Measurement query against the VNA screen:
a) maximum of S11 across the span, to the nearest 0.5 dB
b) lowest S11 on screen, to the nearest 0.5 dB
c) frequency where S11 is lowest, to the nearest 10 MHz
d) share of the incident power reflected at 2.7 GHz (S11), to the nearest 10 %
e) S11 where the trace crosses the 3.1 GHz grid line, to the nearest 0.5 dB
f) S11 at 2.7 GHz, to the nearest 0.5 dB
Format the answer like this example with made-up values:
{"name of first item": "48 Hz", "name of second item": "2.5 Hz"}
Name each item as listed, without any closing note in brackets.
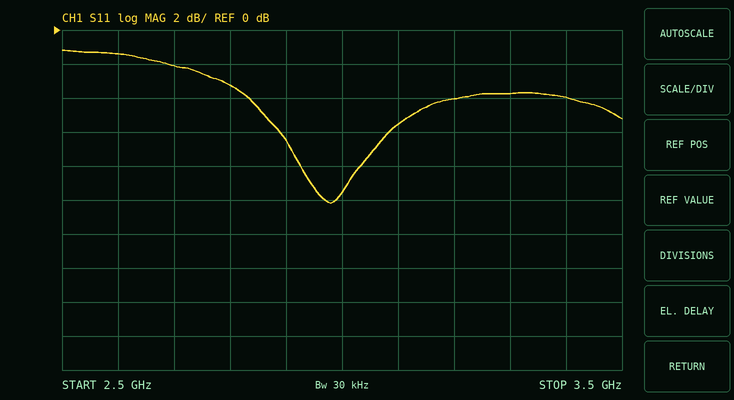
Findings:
{"maximum of S11 across the span, to the nearest 0.5 dB": "-1.0 dB", "lowest S11 on screen, to the nearest 0.5 dB": "-10.0 dB", "frequency where S11 is lowest, to the nearest 10 MHz": "2.98 GHz", "share of the incident power reflected at 2.7 GHz (S11), to the nearest 10 %": "60 %", "S11 where the trace crosses the 3.1 GHz grid line, to the nearest 0.5 dB": "-5.5 dB", "S11 at 2.7 GHz, to the nearest 0.5 dB": "-2.0 dB"}
